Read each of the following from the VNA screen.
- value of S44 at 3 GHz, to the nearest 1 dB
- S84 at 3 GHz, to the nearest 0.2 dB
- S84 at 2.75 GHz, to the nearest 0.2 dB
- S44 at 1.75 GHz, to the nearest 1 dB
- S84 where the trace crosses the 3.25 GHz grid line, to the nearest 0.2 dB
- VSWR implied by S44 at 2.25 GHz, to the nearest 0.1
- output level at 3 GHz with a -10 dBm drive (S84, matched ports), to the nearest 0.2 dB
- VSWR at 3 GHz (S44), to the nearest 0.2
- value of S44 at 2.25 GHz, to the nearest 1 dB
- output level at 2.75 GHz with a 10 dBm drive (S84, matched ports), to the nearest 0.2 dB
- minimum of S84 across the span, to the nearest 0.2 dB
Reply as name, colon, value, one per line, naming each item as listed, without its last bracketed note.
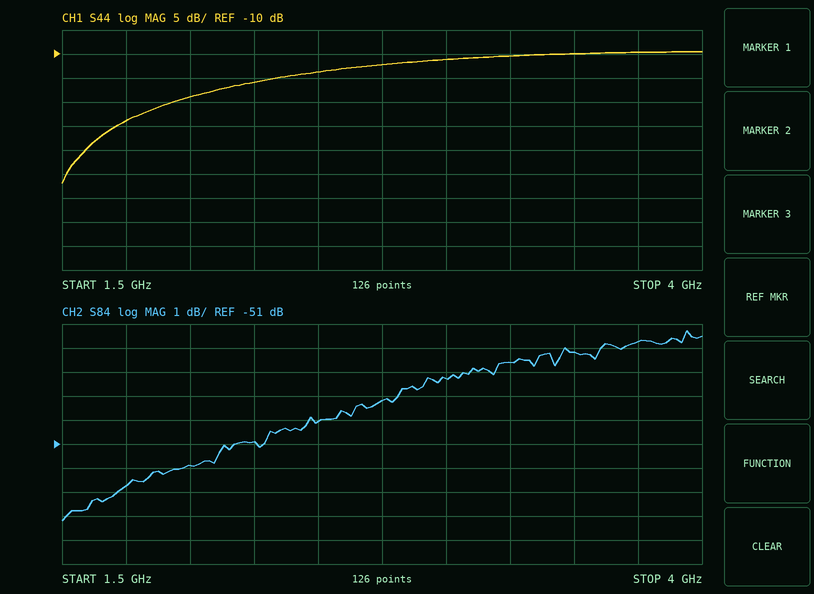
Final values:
value of S44 at 3 GHz, to the nearest 1 dB: -11 dB
S84 at 3 GHz, to the nearest 0.2 dB: -48.2 dB
S84 at 2.75 GHz, to the nearest 0.2 dB: -49.2 dB
S44 at 1.75 GHz, to the nearest 1 dB: -24 dB
S84 where the trace crosses the 3.25 GHz grid line, to the nearest 0.2 dB: -47.6 dB
VSWR implied by S44 at 2.25 GHz, to the nearest 0.1: 1.4
output level at 3 GHz with a -10 dBm drive (S84, matched ports), to the nearest 0.2 dB: -58.2 dBm
VSWR at 3 GHz (S44), to the nearest 0.2: 1.8
value of S44 at 2.25 GHz, to the nearest 1 dB: -16 dB
output level at 2.75 GHz with a 10 dBm drive (S84, matched ports), to the nearest 0.2 dB: -39.2 dBm
minimum of S84 across the span, to the nearest 0.2 dB: -54.2 dB
